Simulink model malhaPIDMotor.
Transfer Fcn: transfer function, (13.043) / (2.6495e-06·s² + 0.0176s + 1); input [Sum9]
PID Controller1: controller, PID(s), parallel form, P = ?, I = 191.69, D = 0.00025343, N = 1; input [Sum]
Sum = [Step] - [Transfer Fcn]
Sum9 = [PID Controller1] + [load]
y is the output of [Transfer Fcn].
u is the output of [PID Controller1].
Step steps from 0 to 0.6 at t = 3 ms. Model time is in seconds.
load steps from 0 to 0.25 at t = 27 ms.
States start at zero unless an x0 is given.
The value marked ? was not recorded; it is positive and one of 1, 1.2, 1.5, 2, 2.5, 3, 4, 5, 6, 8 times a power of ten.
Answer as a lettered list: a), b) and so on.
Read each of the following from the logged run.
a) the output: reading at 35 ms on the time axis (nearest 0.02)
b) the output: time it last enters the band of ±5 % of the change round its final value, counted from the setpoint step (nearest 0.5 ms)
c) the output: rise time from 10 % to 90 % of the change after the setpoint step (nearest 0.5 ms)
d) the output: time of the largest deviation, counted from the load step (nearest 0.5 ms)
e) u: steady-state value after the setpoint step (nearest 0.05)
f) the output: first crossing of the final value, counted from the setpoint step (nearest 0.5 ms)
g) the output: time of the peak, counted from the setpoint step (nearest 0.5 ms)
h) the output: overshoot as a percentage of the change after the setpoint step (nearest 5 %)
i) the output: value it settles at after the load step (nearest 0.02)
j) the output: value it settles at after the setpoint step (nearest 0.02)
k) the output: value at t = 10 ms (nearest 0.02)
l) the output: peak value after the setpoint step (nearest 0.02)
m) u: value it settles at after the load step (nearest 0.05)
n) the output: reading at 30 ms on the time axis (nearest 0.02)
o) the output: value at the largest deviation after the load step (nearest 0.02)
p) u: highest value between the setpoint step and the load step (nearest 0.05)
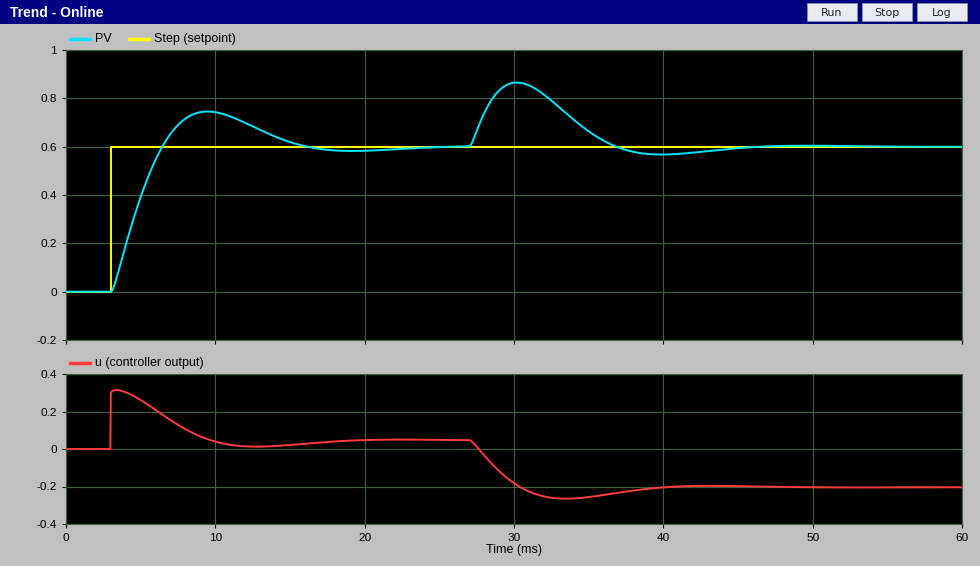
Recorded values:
a) 0.66
b) 11.5 ms
c) 2.5 ms
d) 3.0 ms
e) 0.05
f) 3.5 ms
g) 6.5 ms
h) 25 %
i) 0.60
j) 0.60
k) 0.74
l) 0.74
m) -0.20
n) 0.86
o) 0.86
p) 0.30
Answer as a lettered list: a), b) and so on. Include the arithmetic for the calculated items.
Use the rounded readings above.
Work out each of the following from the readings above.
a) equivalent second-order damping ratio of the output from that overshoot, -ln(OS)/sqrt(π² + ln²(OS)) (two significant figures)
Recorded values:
a) ln(0.25) = -1.386; 1.386 / sqrt(9.870 + 1.922) = 0.40
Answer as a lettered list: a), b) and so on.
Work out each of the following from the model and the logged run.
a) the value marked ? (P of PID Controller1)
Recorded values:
a) 0.5
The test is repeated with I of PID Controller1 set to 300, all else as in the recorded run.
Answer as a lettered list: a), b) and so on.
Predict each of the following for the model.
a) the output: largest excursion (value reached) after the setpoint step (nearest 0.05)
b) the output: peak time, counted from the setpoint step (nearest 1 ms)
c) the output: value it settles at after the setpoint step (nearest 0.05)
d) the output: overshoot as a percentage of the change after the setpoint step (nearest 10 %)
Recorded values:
a) 0.80
b) 5 ms
c) 0.60
d) 30 %
